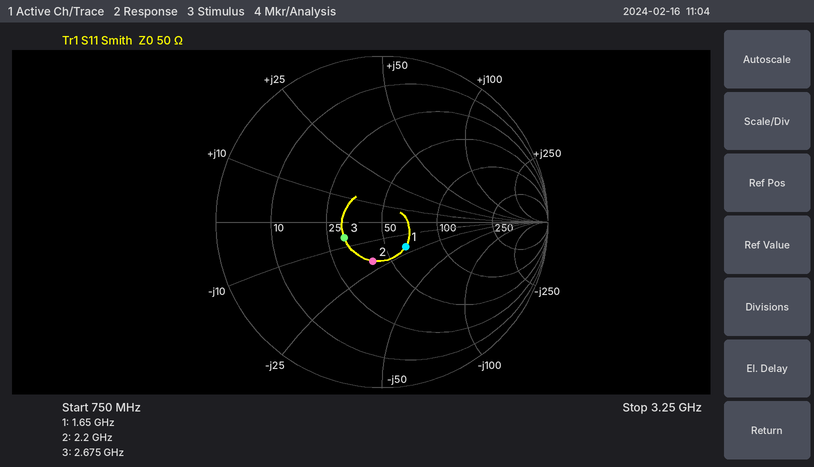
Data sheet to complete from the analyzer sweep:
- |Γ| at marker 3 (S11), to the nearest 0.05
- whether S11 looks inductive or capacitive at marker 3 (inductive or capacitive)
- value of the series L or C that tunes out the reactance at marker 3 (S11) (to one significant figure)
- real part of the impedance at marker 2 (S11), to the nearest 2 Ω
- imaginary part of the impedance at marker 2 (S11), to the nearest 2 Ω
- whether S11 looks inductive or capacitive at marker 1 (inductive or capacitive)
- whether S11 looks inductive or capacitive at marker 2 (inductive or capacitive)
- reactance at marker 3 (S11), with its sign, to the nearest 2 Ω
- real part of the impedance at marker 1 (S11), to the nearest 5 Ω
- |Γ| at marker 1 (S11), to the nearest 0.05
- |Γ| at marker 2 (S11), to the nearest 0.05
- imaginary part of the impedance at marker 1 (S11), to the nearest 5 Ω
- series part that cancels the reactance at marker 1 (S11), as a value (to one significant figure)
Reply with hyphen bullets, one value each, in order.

- 0.25
- capacitive
- 400 pH
- 40 Ω
- -20 Ω
- capacitive
- capacitive
- -6 Ω
- 65 Ω
- 0.20
- 0.25
- -20 Ω
- 2 nH
